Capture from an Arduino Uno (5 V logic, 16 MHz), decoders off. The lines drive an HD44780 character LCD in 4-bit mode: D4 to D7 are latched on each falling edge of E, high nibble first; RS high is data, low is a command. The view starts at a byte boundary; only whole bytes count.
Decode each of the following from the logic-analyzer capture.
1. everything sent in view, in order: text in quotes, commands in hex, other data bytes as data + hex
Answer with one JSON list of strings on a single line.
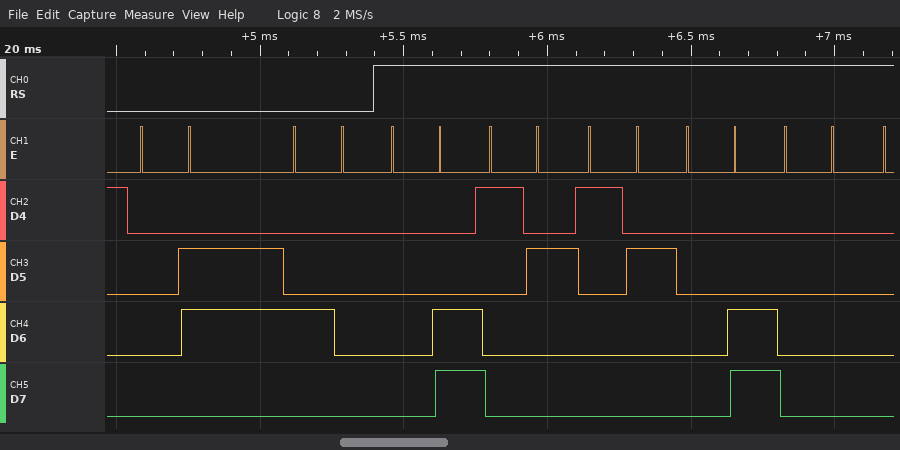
["0x06 0x40 data 0C 12 12 0C 00"]
